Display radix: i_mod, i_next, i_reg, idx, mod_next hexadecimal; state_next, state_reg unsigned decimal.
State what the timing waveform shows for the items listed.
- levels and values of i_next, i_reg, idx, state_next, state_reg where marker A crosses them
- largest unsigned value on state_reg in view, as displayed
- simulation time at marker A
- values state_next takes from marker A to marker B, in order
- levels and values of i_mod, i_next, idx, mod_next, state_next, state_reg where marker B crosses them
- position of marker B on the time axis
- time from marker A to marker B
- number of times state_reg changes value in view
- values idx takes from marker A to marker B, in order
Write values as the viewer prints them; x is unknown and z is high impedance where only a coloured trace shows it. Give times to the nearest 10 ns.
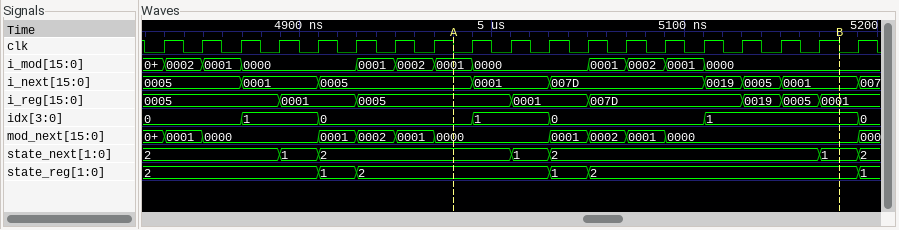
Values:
i_next=0005, i_reg=0005, idx=0, state_next=2, state_reg=2
2
4980 ns
2, 1, 2, 1
i_mod=0000, i_next=0001, idx=1, mod_next=0000, state_next=1, state_reg=2
5180 ns
200 ns
5
0, 1, 0, 1
